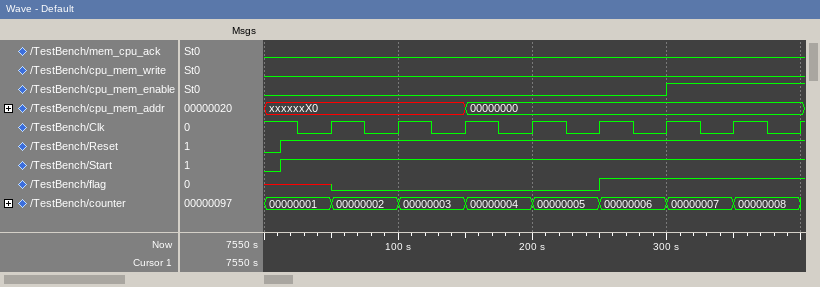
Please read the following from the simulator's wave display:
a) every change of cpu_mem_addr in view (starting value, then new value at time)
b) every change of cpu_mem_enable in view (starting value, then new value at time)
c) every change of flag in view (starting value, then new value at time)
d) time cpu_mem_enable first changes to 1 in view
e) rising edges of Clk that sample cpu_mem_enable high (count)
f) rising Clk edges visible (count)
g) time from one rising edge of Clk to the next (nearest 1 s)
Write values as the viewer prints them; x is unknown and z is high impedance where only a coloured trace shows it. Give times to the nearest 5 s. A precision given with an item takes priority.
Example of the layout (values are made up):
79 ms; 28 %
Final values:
xxxxxxX0, 00000000 at 150 s; 0, 1 at 300 s; x, 0 at 50 s, 1 at 250 s; 300 s; 2; 8; 50 s
